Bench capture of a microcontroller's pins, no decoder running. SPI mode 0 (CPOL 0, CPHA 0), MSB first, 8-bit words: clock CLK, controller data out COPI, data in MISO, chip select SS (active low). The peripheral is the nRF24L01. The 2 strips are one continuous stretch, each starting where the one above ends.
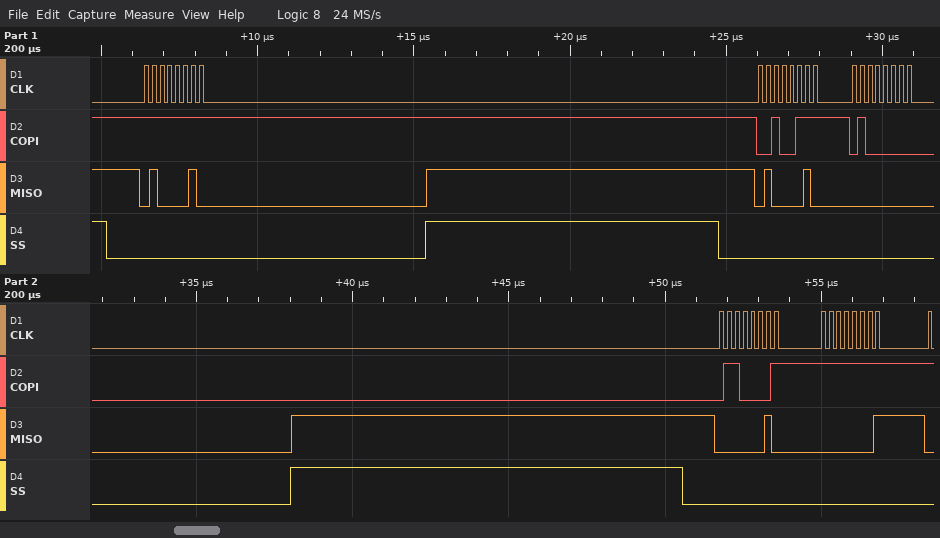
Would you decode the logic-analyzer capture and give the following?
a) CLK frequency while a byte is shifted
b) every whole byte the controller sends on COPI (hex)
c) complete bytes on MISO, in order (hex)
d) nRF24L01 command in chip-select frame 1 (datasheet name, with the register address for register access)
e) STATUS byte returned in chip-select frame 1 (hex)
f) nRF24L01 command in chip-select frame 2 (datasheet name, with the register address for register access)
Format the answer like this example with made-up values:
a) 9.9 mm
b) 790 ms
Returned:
a) 4 MHz
b) 0xFF 0x27 0x40 0x61 0xFF
c) 0x42 0x42 0x00 0x02 0x01
d) NOP
e) 0x42
f) W_REGISTER 0x07
